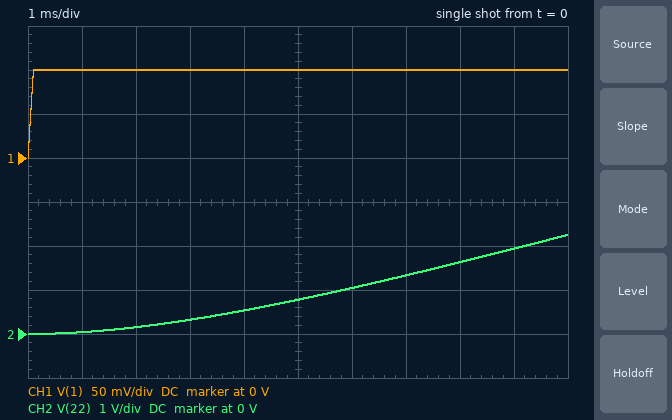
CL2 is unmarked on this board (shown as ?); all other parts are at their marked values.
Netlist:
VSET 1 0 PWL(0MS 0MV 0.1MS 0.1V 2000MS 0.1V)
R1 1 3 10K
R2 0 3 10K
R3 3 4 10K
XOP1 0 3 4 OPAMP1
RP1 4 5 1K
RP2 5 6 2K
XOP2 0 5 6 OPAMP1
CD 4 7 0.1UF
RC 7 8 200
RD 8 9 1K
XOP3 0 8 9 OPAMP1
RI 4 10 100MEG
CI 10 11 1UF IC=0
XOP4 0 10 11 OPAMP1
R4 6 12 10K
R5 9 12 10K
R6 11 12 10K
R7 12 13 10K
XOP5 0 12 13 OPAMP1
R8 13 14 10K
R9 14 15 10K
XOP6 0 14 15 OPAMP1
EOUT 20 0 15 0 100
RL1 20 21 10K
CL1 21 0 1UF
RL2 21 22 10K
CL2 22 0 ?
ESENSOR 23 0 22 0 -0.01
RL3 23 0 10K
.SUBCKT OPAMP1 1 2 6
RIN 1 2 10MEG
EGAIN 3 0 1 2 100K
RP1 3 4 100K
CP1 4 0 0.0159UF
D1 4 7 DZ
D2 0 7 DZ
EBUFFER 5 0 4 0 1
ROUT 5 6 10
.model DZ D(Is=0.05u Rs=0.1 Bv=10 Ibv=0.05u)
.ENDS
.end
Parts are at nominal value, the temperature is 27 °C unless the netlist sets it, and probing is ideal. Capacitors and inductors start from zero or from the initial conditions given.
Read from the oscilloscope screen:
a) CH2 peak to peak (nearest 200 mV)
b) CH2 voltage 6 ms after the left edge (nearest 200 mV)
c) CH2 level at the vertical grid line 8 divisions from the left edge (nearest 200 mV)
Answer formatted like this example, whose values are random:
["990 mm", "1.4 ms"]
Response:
["2.2 V", "1.0 V", "1.6 V"]
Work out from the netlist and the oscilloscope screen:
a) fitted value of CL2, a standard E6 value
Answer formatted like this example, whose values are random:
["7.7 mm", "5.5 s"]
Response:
["2.2 µF"]
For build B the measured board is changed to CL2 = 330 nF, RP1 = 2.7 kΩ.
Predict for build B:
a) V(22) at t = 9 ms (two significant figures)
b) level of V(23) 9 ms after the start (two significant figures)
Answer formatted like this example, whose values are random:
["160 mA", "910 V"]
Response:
["2.8 V", "-28 mV"]
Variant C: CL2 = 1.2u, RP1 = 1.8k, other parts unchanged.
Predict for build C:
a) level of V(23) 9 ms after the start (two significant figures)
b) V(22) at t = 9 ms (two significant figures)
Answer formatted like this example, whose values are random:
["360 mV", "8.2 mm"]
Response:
["-18 mV", "1.8 V"]
